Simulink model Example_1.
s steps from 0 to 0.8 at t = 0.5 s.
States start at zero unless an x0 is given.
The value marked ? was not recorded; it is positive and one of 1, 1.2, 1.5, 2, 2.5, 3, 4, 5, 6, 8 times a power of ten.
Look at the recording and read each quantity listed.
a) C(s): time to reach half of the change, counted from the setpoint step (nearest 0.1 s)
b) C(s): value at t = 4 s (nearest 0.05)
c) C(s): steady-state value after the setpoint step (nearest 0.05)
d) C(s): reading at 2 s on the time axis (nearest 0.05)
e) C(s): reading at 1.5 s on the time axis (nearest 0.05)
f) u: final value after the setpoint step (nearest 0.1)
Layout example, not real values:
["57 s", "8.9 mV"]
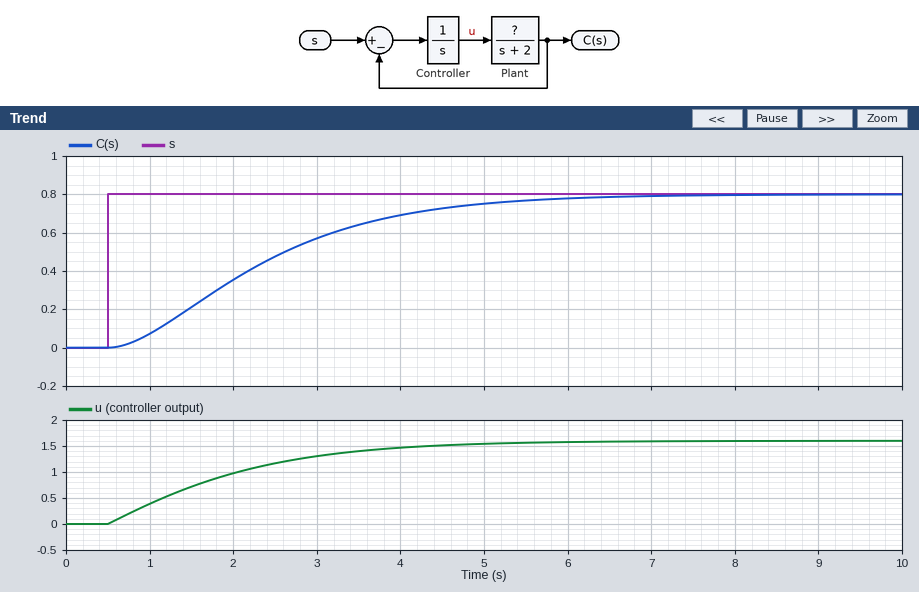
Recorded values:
["1.7 s", "0.70", "0.80", "0.35", "0.20", "1.6"]
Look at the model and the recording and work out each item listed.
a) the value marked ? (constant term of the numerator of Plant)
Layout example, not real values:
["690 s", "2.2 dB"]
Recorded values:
["1"]
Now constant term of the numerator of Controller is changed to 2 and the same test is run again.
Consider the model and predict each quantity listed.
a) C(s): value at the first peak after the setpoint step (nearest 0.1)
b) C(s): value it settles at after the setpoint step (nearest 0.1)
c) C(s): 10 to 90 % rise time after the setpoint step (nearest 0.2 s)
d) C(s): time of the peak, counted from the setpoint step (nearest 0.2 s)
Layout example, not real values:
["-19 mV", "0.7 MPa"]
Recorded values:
["0.8", "0.8", "1.6 s", "3.2 s"]
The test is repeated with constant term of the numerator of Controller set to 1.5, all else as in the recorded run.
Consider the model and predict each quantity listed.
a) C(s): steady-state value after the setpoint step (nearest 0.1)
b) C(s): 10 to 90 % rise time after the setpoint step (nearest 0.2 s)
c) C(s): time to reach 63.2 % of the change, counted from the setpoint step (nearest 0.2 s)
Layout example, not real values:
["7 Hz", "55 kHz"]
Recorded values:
["0.8", "2.0 s", "1.6 s"]
